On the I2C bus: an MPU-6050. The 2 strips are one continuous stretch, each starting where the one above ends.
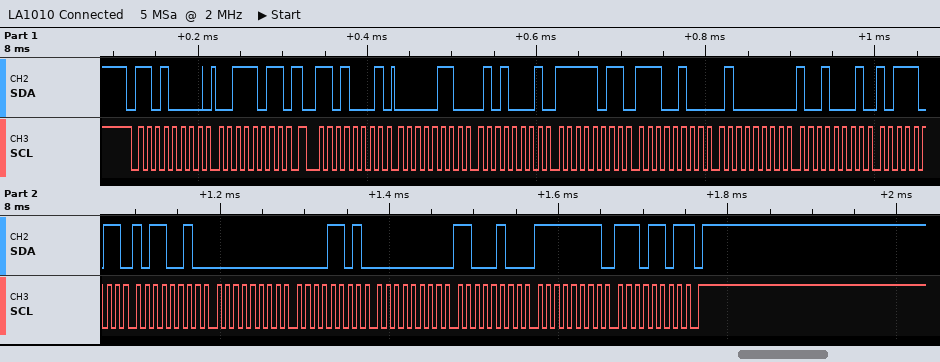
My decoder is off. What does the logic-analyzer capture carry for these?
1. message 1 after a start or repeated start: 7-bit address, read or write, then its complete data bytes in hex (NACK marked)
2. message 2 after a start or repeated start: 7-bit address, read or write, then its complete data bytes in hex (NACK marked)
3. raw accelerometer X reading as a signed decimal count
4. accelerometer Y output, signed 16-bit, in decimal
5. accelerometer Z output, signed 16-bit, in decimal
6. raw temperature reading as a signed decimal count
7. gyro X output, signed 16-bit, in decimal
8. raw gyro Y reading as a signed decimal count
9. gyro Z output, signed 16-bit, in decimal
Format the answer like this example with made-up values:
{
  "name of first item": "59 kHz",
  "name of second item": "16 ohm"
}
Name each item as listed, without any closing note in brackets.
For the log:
{
  "message 1 after a start or repeated start: 7-bit address, read or write, then its complete data bytes in hex": "0x68 write: 3B",
  "message 2 after a start or repeated start: 7-bit address, read or write, then its complete data bytes in hex": "0x68 read: 06 51 FB E4 40 91 BB B2 00 0D 00 C4 FF ED NACK",
  "raw accelerometer X reading as a signed decimal count": "1617",
  "accelerometer Y output, signed 16-bit, in decimal": "-1052",
  "accelerometer Z output, signed 16-bit, in decimal": "16529",
  "raw temperature reading as a signed decimal count": "-17486",
  "gyro X output, signed 16-bit, in decimal": "13",
  "raw gyro Y reading as a signed decimal count": "196",
  "gyro Z output, signed 16-bit, in decimal": "-19"
}
